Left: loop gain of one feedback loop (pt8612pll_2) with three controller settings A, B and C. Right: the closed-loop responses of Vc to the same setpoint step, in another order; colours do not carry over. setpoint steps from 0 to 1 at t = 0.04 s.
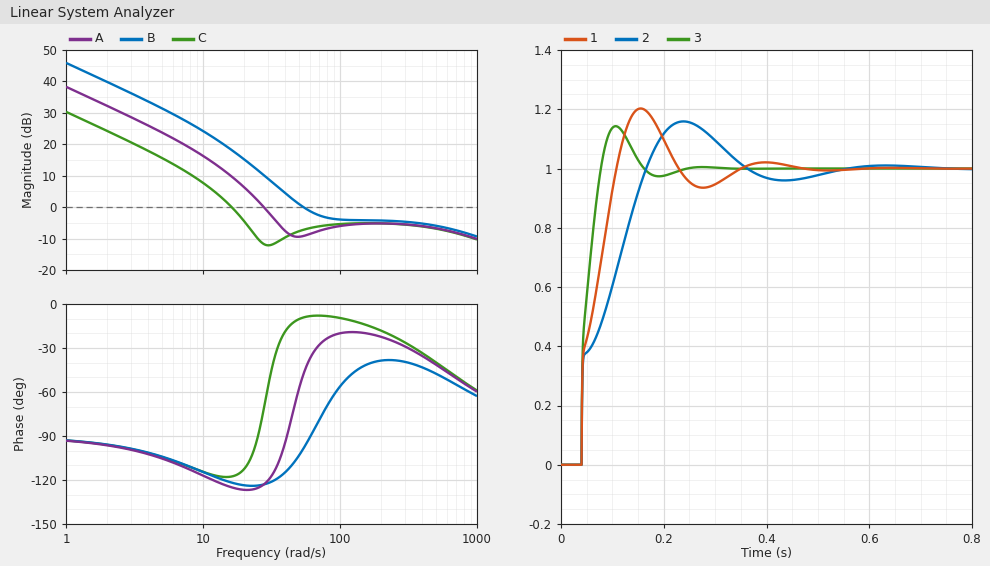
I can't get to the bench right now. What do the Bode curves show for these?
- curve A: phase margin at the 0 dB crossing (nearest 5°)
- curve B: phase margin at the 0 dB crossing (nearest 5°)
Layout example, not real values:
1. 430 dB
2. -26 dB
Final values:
1. 55°
2. 80°
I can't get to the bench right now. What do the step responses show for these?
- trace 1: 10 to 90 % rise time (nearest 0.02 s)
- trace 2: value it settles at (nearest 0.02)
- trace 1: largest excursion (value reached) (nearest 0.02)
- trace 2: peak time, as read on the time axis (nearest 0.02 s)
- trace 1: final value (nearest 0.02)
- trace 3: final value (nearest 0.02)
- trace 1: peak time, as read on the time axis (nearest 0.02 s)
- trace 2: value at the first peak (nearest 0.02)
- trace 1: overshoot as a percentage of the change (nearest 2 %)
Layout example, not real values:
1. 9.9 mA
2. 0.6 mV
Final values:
1. 0.06 s
2. 1.00
3. 1.20
4. 0.24 s
5. 1.00
6. 1.00
7. 0.16 s
8. 1.16
9. 20 %
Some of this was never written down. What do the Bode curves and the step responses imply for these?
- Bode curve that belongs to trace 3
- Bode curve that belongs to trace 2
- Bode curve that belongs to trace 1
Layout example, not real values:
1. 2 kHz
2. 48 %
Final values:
1. B
2. C
3. A
